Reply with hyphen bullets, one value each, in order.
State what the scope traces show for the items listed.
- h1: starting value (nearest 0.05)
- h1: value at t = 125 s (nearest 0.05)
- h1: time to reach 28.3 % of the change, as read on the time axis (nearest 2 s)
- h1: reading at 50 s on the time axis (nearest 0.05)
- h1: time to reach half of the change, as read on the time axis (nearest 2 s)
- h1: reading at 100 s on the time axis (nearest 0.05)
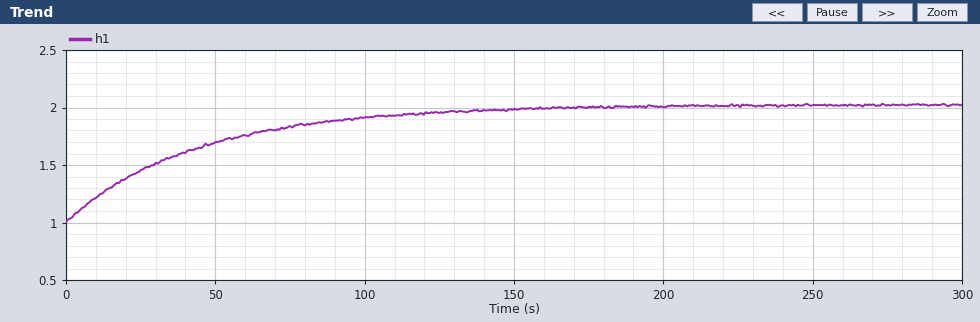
- 1.00
- 1.95
- 14 s
- 1.70
- 30 s
- 1.90
